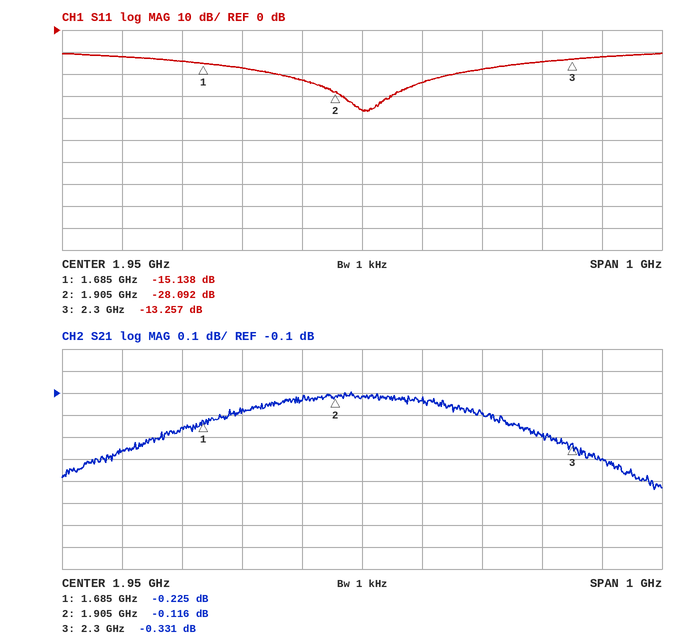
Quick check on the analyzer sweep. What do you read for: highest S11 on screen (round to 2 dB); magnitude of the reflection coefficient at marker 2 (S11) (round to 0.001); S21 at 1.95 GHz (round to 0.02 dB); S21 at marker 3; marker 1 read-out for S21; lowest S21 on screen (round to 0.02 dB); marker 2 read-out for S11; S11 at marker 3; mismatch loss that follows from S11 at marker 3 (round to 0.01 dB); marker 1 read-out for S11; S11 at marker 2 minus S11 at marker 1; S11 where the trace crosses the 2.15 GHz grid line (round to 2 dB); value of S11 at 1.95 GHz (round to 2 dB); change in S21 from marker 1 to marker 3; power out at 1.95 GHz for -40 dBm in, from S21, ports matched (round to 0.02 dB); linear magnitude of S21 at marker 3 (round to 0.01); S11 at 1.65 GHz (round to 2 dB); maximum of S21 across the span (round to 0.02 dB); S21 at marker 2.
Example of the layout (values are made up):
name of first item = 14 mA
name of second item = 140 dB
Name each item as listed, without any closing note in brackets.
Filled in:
highest S11 on screen = -10 dB
magnitude of the reflection coefficient at marker 2 (S11) = 0.039
S21 at 1.95 GHz = -0.12 dB
S21 at marker 3 = -0.331 dB
marker 1 read-out for S21 = -0.225 dB
lowest S21 on screen = -0.54 dB
marker 2 read-out for S11 = -28.092 dB
S11 at marker 3 = -13.257 dB
mismatch loss that follows from S11 at marker 3 = 0.21 dB
marker 1 read-out for S11 = -15.138 dB
S11 at marker 2 minus S11 at marker 1 = -12.954 dB
S11 where the trace crosses the 2.15 GHz grid line = -18 dB
value of S11 at 1.95 GHz = -36 dB
change in S21 from marker 1 to marker 3 = -0.106 dB
power out at 1.95 GHz for -40 dBm in, from S21, ports matched = -40.12 dBm
linear magnitude of S21 at marker 3 = 0.96
S11 at 1.65 GHz = -14 dB
maximum of S21 across the span = -0.10 dB
S21 at marker 2 = -0.116 dB
